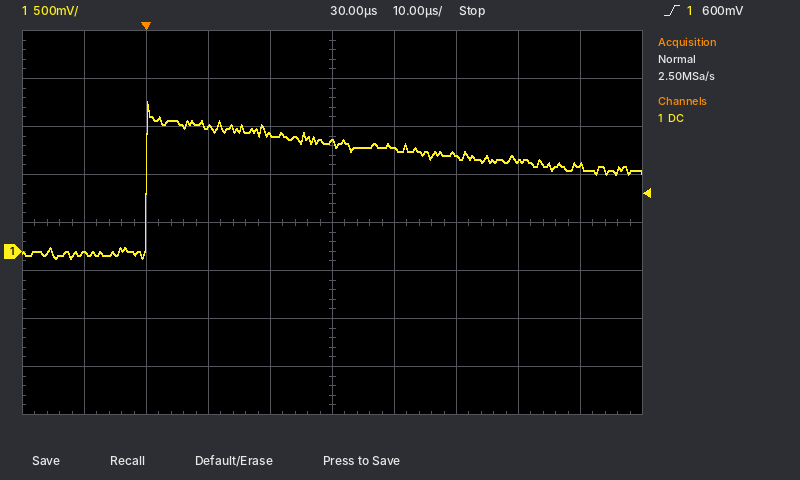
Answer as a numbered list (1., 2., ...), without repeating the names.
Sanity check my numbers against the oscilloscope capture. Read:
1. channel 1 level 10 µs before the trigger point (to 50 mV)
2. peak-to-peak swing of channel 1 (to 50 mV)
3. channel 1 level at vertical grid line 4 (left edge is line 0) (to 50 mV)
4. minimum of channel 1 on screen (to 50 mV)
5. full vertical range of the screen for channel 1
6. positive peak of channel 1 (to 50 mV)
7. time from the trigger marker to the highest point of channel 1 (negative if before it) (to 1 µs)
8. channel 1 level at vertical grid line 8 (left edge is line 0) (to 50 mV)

1. 0 mV
2. 1.65 V
3. 1.20 V
4. -100 mV
5. 4 V
6. 1.55 V
7. 0 µs
8. 950 mV
